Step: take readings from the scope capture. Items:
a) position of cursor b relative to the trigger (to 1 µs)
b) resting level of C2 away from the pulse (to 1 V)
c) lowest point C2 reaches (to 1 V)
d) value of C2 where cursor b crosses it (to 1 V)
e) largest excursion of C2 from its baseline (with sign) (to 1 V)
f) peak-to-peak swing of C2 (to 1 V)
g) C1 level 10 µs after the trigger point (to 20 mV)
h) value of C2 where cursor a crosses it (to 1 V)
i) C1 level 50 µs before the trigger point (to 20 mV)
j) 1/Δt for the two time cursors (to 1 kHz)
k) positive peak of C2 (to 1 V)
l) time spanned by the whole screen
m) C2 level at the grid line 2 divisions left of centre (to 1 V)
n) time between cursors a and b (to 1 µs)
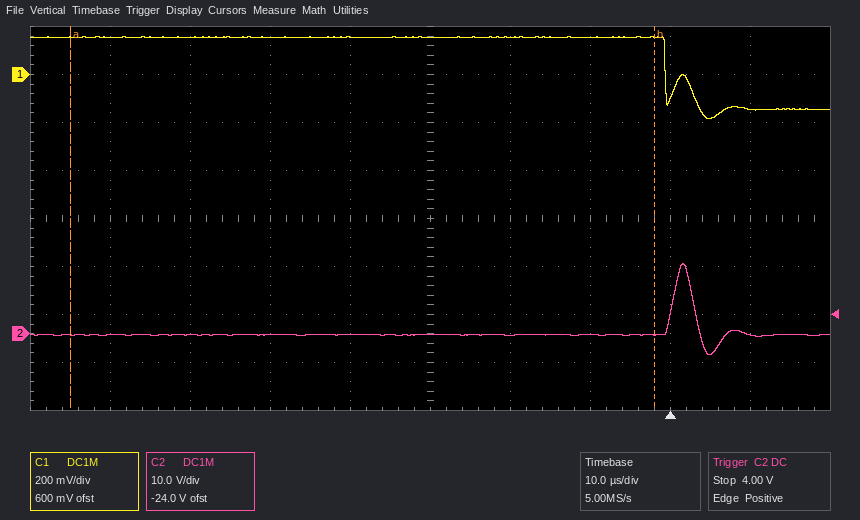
-2 µs
0 V
-4 V
0 V
+15 V
19 V
-140 mV
0 V
160 mV
14 kHz
15 V
100 µs
0 V
73 µs
